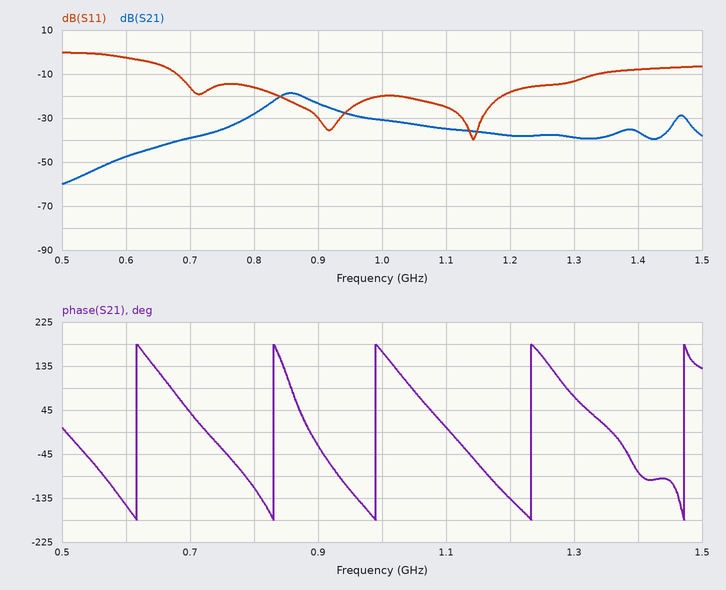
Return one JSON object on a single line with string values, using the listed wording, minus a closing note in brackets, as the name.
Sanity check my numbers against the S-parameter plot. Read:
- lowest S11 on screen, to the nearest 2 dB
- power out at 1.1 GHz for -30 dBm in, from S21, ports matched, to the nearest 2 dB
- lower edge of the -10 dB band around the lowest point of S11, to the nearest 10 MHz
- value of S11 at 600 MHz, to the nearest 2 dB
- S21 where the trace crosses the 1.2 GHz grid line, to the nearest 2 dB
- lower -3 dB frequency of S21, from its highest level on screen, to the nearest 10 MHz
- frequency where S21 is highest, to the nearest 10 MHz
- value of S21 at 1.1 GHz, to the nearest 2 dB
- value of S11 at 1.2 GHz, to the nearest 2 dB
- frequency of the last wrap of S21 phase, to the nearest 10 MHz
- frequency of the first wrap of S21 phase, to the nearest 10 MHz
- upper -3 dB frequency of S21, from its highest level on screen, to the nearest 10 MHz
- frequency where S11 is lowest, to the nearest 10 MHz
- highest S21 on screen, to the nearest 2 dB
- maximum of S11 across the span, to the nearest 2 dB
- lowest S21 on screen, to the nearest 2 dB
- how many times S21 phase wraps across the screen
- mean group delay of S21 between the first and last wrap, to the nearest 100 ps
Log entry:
{"lowest S11 on screen, to the nearest 2 dB": "-40 dB", "power out at 1.1 GHz for -30 dBm in, from S21, ports matched, to the nearest 2 dB": "-64 dBm", "lower edge of the -10 dB band around the lowest point of S11, to the nearest 10 MHz": "680 MHz", "value of S11 at 600 MHz, to the nearest 2 dB": "-2 dB", "S21 where the trace crosses the 1.2 GHz grid line, to the nearest 2 dB": "-38 dB", "lower -3 dB frequency of S21, from its highest level on screen, to the nearest 10 MHz": "830 MHz", "frequency where S21 is highest, to the nearest 10 MHz": "860 MHz", "value of S21 at 1.1 GHz, to the nearest 2 dB": "-34 dB", "value of S11 at 1.2 GHz, to the nearest 2 dB": "-18 dB", "frequency of the last wrap of S21 phase, to the nearest 10 MHz": "1.47 GHz", "frequency of the first wrap of S21 phase, to the nearest 10 MHz": "620 MHz", "upper -3 dB frequency of S21, from its highest level on screen, to the nearest 10 MHz": "890 MHz", "frequency where S11 is lowest, to the nearest 10 MHz": "1.14 GHz", "highest S21 on screen, to the nearest 2 dB": "-18 dB", "maximum of S11 across the span, to the nearest 2 dB": "0 dB", "lowest S21 on screen, to the nearest 2 dB": "-60 dB", "how many times S21 phase wraps across the screen": "5", "mean group delay of S21 between the first and last wrap, to the nearest 100 ps": "4.7 ns"}
